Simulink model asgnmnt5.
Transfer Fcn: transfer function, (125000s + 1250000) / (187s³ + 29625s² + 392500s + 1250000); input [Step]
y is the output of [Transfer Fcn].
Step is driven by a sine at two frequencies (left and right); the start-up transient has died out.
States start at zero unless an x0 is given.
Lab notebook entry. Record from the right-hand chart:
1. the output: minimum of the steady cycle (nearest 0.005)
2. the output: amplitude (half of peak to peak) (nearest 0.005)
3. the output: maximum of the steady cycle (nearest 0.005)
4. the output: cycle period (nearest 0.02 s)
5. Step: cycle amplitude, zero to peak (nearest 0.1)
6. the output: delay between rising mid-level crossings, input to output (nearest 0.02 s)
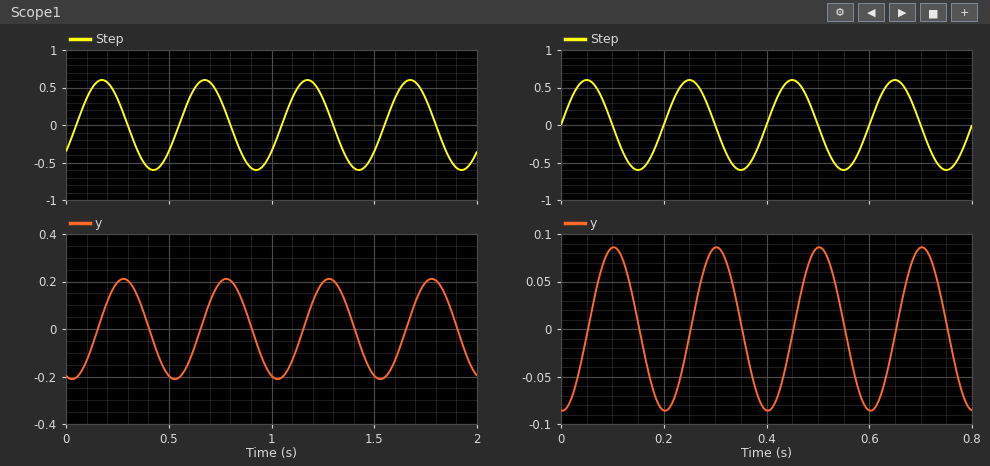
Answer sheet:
-0.085
0.085
0.085
0.20 s
0.6
0.06 s
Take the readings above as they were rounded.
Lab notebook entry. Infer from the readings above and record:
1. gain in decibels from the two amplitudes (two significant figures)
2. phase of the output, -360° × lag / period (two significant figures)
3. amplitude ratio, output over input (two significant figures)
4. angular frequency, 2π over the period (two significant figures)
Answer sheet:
-17 dB
-110°
0.14
31 rad/s
